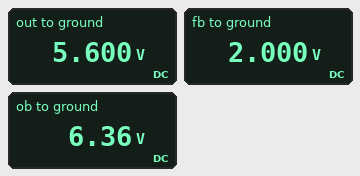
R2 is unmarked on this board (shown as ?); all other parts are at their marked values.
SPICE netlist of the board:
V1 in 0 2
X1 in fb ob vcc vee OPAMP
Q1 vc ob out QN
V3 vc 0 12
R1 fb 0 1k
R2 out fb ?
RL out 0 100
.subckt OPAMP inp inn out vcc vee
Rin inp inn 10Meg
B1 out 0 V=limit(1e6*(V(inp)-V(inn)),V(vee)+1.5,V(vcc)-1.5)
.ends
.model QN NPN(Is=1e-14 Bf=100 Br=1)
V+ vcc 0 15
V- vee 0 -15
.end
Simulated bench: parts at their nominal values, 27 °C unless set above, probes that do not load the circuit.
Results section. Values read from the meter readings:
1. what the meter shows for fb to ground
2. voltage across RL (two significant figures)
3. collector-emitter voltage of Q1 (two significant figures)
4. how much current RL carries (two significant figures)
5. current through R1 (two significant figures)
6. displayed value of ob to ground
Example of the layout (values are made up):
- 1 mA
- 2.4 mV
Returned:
- 2.000 V
- 5.6 V
- 6.4 V
- 56 mA
- 2.0 mA
- 6.36 V
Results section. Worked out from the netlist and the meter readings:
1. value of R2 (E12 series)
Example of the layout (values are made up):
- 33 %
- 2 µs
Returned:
- 1.8 kΩ
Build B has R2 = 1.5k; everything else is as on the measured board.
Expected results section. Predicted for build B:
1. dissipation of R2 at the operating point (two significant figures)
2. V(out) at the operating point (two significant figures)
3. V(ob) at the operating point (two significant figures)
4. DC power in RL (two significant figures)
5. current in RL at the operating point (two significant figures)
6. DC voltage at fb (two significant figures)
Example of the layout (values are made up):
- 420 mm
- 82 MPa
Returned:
- 6.0 mW
- 5.0 V
- 5.8 V
- 250 mW
- 50 mA
- 2.0 V
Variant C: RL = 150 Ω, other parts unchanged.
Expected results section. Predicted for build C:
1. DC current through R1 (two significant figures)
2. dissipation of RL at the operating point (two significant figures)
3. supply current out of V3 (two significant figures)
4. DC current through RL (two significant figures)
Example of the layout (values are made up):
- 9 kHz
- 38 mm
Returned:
- 2.0 mA
- 210 mW
- 39 mA
- 37 mA
